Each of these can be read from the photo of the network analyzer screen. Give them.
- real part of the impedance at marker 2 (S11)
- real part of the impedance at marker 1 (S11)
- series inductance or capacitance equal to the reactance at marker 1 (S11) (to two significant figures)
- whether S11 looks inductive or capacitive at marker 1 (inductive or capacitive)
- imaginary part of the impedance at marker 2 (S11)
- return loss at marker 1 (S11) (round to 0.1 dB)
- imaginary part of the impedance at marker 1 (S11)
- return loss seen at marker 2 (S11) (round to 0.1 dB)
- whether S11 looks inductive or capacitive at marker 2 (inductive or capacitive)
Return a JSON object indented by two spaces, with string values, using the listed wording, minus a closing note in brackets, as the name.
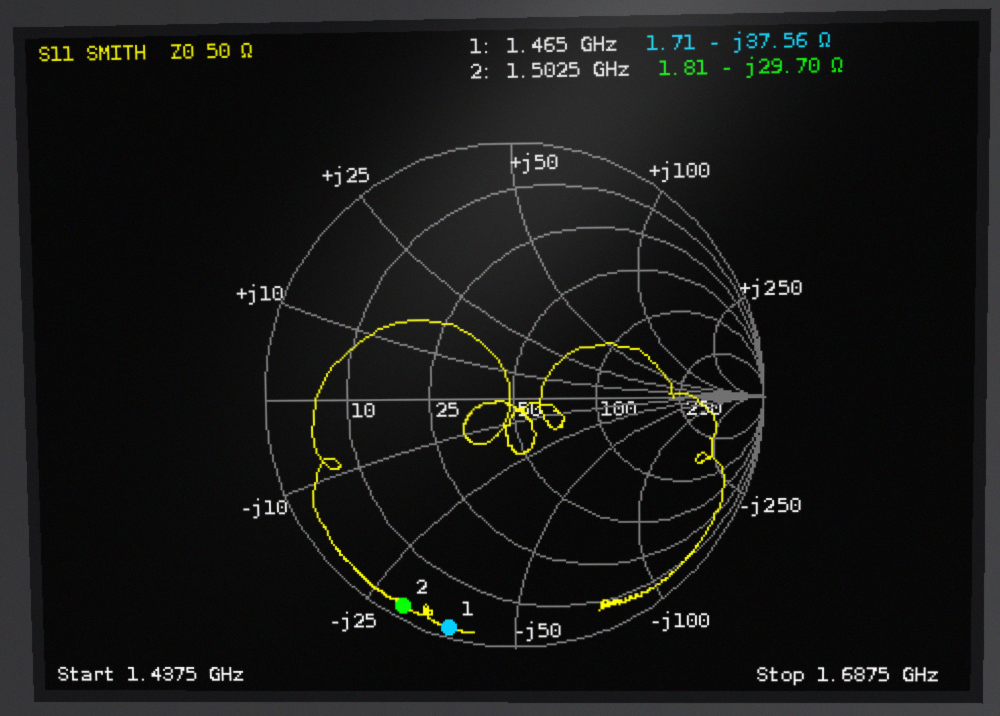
{
  "real part of the impedance at marker 2": "1.81 Ω",
  "real part of the impedance at marker 1": "1.71 Ω",
  "series inductance or capacitance equal to the reactance at marker 1 (S11)": "2.9 pF",
  "whether S11 looks inductive or capacitive at marker 1": "capacitive",
  "imaginary part of the impedance at marker 2": "-29.70 Ω",
  "return loss at marker 1 (S11)": "0.4 dB",
  "imaginary part of the impedance at marker 1": "-37.56 Ω",
  "return loss seen at marker 2 (S11)": "0.5 dB",
  "whether S11 looks inductive or capacitive at marker 2": "capacitive"
}
